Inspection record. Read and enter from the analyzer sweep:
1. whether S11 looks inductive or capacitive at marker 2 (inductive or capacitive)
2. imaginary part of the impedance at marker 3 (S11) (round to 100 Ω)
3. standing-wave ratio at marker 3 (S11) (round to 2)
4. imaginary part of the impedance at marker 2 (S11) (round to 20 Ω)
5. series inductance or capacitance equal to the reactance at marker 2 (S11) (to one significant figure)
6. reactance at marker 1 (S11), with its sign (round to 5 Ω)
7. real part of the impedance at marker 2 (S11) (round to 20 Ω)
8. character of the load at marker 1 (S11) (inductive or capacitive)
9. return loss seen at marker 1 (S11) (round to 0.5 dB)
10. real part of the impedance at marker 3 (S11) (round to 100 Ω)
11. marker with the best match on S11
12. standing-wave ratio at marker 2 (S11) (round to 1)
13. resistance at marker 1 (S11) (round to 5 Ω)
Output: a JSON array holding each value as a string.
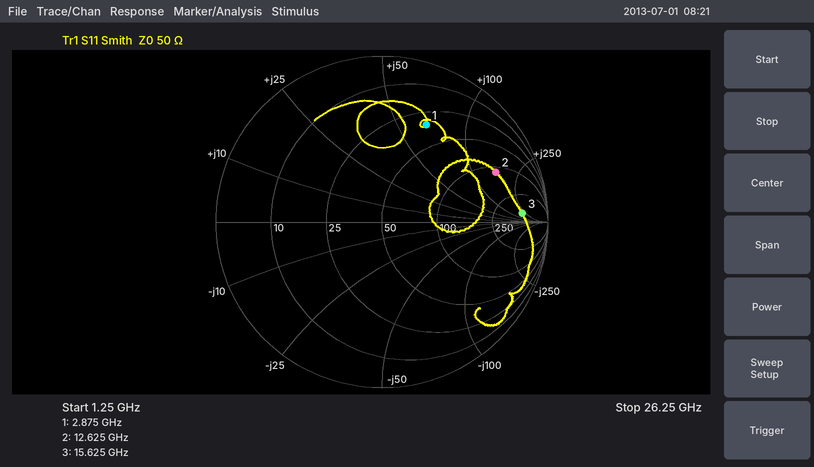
["inductive", "+200 Ω", "12", "+160 Ω", "2 nH", "+65 Ω", "120 Ω", "inductive", "4.0 dB", "500 Ω", "marker 1", "7", "35 Ω"]
